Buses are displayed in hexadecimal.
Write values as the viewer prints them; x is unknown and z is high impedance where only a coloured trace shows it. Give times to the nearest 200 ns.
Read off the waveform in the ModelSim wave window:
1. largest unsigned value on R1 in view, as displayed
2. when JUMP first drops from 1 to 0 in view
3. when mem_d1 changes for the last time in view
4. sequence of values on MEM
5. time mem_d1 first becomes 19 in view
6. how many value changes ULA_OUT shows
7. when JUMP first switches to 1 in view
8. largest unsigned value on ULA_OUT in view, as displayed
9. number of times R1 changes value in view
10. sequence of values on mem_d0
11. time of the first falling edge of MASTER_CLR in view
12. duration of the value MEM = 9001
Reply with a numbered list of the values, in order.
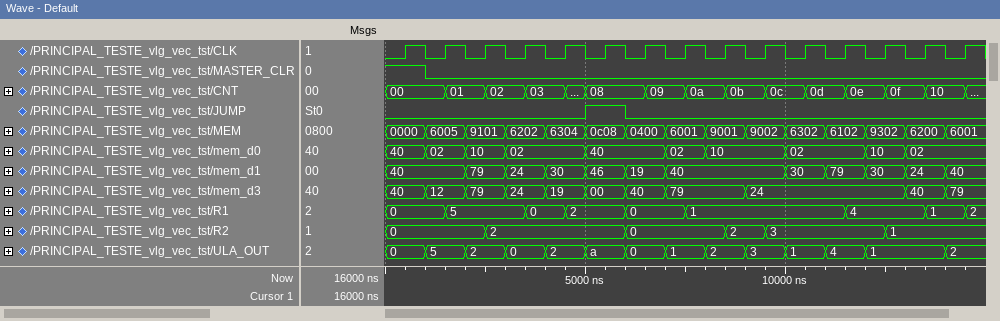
1. 5
2. 6000 ns
3. 14000 ns
4. 0000, 6005, 9101, 6202, 6304, 0c08, 0400, 6001, 9001, 9002, 6302, 6102, 9302, 6200, 6001
5. 6000 ns
6. 13
7. 5000 ns
8. a
9. 8
10. 40, 02, 10, 02, 40, 02, 10, 02, 10, 02
11. 1000 ns
12. 1000 ns
